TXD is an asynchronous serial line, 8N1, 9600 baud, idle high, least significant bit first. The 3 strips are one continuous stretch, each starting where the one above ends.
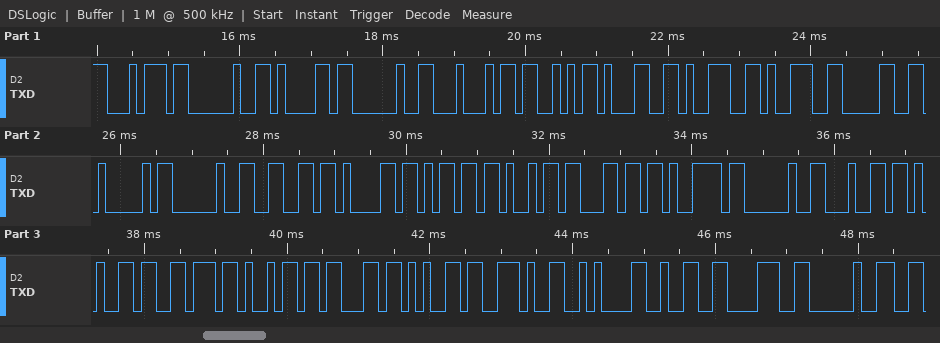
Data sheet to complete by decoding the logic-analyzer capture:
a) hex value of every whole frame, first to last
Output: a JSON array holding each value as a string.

["0x74 0x20 0x61 0x20 0x44 0x53 0x31 0x39 0x39 0x30 0x41 0x20 0x66 0x61 0x6D 0x69 0x6C 0x79 0x20 0x64 0x65 0x76 0x69 0x63 0x65 0x2E 0x0A 0x32 0x38 0x20"]
